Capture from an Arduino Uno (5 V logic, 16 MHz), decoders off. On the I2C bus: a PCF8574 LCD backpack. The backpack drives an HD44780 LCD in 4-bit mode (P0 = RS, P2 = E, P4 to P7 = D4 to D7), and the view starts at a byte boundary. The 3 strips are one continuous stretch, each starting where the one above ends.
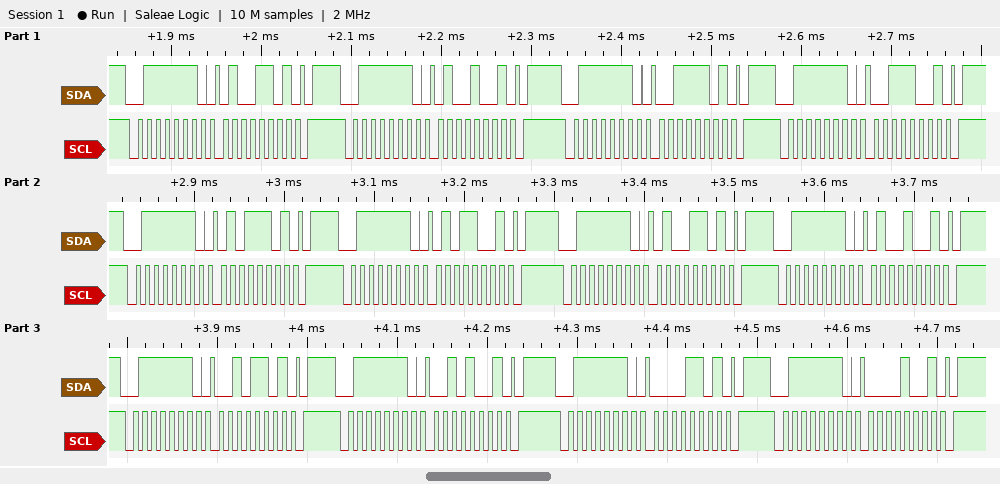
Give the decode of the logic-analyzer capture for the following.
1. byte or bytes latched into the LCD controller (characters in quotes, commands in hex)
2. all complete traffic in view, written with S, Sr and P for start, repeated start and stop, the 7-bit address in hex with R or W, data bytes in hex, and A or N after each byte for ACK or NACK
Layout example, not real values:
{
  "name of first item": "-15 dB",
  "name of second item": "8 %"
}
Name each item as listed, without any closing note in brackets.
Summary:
{
  "byte or bytes latched into the LCD controller": "'C' 'T' ' '",
  "all complete traffic in view, written with S, Sr and P for start, repeated start and stop, the 7-bit address in hex with R or W, data bytes in hex, and A or N after each byte for ACK or NACK": "S 3FW A 4D A P S 3FW A 49 A P S 3FW A 3D A P S 3FW A 39 A P S 3FW A 5D A P S 3FW A 59 A P S 3FW A 4D A P S 3FW A 49 A P S 3FW A 2D A P S 3FW A 29 A P S 3FW A 0D A P S 3FW A 09 A P"
}
